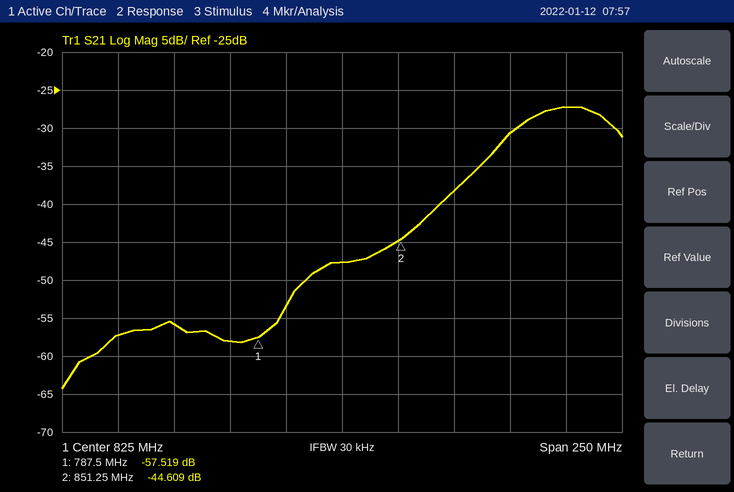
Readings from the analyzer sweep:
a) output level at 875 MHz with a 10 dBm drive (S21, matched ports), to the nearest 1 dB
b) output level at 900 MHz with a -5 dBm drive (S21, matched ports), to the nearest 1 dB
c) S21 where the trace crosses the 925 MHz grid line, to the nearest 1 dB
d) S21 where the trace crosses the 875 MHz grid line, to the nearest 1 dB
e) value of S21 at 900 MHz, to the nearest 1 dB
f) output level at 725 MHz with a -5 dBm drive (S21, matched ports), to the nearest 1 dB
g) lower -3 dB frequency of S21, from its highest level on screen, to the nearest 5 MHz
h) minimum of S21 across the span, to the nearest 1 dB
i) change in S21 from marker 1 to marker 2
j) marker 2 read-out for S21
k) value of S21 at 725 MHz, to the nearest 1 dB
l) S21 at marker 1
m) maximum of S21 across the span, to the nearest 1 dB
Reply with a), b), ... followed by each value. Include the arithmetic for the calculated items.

a) 10 dBm + (-38 dB) = -28 dBm
b) -5 dBm + (-31 dB) = -36 dBm
c) -27 dB
d) -38 dB
e) -31 dB
f) -5 dBm + (-57 dB) = -62 dBm
g) 900 MHz
h) -64 dB
i) -44.609 − (-57.519) = 12.910 dB
j) -44.609 dB
k) -57 dB
l) -57.519 dB
m) -27 dB
